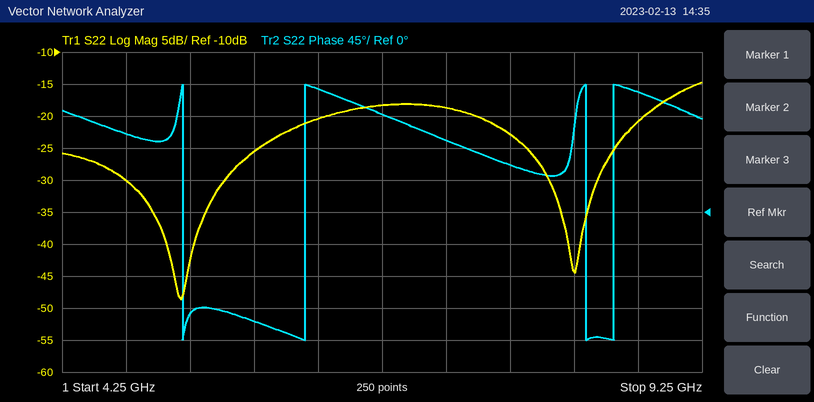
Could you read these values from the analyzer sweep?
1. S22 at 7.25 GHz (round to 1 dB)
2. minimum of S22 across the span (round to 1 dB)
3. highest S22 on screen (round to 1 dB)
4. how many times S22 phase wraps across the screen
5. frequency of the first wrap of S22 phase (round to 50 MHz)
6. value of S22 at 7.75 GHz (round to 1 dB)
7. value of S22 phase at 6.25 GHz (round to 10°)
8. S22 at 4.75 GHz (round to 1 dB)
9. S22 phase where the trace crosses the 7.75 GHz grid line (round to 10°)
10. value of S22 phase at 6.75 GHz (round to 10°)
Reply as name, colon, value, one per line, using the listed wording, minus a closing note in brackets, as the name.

S22 at 7.25 GHz: -19 dB
minimum of S22 across the span: -49 dB
highest S22 on screen: -15 dB
how many times S22 phase wraps across the screen: 4
frequency of the first wrap of S22 phase: 5.20 GHz
value of S22 at 7.75 GHz: -23 dB
value of S22 phase at 6.25 GHz: 170°
S22 at 4.75 GHz: -30 dB
S22 phase where the trace crosses the 7.75 GHz grid line: 70°
value of S22 phase at 6.75 GHz: 140°
